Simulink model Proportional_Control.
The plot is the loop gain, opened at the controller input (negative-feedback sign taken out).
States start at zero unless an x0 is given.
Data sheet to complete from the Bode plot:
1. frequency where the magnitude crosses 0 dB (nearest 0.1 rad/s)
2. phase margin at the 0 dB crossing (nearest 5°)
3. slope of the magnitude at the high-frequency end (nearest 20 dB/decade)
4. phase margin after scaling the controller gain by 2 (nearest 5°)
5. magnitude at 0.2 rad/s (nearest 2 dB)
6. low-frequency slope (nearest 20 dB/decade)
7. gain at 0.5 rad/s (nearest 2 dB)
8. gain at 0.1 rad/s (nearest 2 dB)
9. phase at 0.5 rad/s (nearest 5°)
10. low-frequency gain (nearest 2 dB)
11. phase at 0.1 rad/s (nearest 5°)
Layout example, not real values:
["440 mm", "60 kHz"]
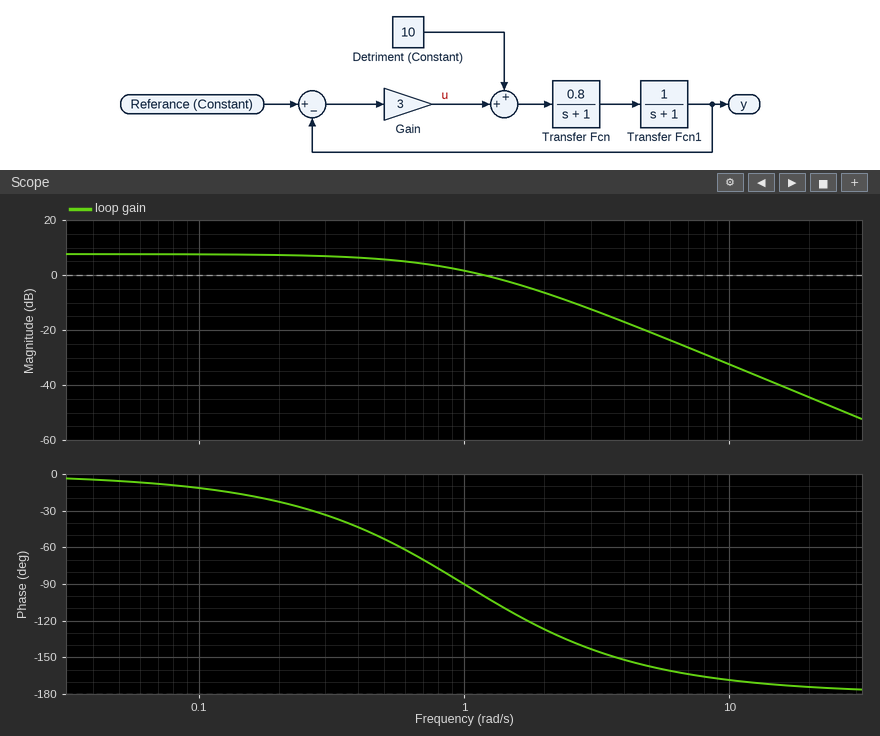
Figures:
["1.2 rad/s", "80°", "-40 dB/decade", "55°", "8 dB", "0 dB/decade", "6 dB", "8 dB", "-55°", "8 dB", "-10°"]
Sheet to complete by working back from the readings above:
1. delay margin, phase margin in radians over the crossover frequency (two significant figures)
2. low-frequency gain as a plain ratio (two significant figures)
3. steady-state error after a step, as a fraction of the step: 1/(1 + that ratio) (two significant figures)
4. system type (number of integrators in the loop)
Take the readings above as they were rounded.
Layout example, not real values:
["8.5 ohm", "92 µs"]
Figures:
["1.2 s", "2.5", "0.29", "0"]
